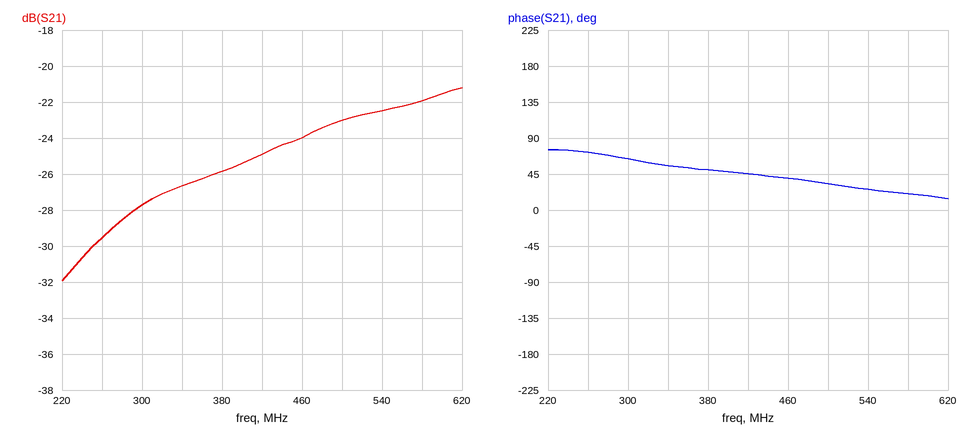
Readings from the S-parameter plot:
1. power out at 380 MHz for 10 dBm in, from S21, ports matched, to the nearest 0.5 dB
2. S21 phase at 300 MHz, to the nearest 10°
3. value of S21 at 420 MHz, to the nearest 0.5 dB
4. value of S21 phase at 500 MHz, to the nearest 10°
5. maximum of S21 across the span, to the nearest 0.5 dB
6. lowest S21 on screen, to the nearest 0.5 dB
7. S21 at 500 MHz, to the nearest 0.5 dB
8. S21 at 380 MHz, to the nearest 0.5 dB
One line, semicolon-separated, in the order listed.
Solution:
-16.0 dBm; 60°; -25.0 dB; 30°; -21.0 dB; -32.0 dB; -23.0 dB; -26.0 dB
